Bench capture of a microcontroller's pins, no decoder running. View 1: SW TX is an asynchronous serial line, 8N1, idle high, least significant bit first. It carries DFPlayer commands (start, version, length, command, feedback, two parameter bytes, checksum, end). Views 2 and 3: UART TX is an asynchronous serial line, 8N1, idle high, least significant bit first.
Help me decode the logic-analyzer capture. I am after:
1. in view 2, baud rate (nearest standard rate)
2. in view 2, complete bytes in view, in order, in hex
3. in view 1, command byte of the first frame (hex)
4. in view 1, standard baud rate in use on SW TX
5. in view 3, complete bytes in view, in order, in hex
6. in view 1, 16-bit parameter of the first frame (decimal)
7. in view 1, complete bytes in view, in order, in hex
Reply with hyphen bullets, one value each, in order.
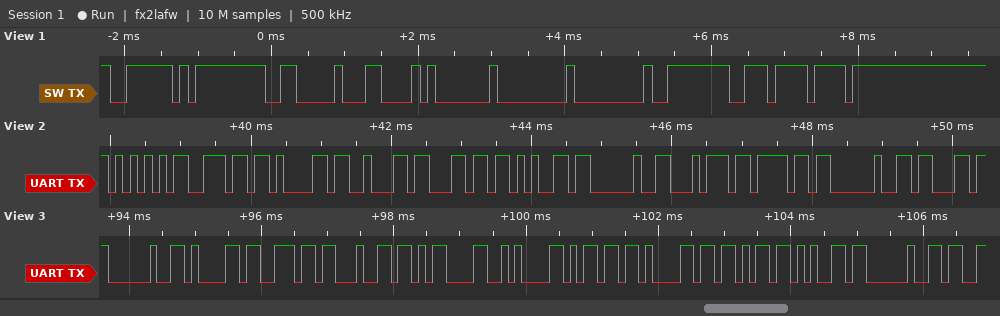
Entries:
- 9600 baud
- 0x55 0x6E 0x61 0x62 0x6C 0x65 0x20 0x74 0x6F 0x20 0x63
- 0x0C
- 9600 baud
- 20 61 6E 64 0D 0A 6D 61 6B 65 20
- 0
- 0x7E 0xFF 0x06 0x0C 0x01 0x00 0x00 0xFE 0xEE 0xEF
